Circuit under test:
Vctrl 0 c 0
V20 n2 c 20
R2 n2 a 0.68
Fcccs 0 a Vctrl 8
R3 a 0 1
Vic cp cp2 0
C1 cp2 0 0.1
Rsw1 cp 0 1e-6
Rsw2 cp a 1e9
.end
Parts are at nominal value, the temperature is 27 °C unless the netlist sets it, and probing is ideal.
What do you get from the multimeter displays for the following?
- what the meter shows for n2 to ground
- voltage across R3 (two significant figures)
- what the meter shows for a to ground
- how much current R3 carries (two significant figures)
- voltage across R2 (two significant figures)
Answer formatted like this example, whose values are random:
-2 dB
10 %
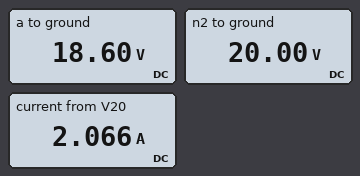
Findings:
20.00 V
19 V
18.60 V
19 A
1.4 V
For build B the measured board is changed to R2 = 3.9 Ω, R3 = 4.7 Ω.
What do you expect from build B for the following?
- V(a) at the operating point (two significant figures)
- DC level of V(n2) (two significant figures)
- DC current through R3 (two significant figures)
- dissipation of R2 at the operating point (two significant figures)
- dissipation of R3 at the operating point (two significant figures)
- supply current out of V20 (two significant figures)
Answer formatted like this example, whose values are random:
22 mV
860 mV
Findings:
18 V
20 V
3.9 A
730 mW
71 W
430 mA
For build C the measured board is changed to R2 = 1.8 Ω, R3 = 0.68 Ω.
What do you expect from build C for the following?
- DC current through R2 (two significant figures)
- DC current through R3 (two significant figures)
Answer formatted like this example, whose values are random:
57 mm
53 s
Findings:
2.5 A
23 A
